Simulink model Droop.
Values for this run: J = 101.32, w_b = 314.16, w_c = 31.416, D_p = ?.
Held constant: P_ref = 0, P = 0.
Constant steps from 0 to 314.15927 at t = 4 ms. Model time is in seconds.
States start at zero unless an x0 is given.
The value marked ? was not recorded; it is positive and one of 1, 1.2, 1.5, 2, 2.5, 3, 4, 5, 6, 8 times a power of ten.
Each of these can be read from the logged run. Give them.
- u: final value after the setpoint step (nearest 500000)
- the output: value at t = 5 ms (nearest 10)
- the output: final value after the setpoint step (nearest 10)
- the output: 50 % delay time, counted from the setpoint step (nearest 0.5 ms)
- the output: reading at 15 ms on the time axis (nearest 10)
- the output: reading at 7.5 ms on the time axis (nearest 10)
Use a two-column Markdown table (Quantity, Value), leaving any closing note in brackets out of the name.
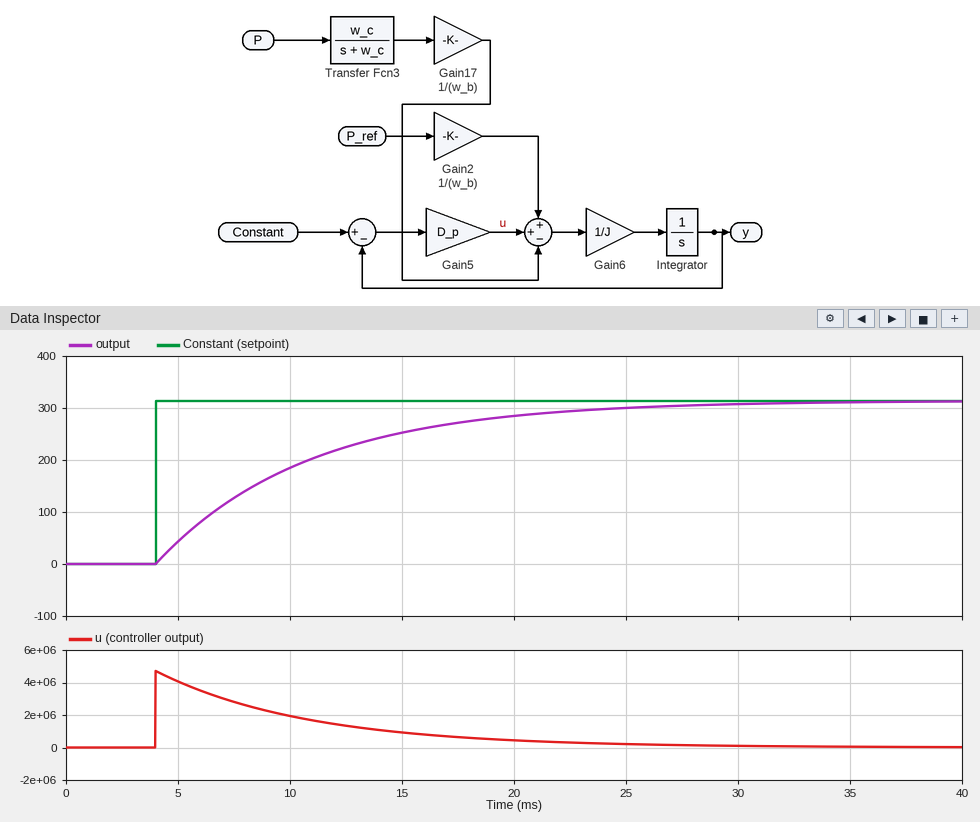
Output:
| Quantity | Value |
|---|---|
| u: final value after the setpoint step | 0 |
| the output: value at t = 5 ms | 40 |
| the output: final value after the setpoint step | 310 |
| the output: 50 % delay time, counted from the setpoint step | 4.5 ms |
| the output: reading at 15 ms on the time axis | 250 |
| the output: reading at 7.5 ms on the time axis | 130 |
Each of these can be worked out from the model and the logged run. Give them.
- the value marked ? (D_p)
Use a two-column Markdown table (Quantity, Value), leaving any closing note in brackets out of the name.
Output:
| Quantity | Value |
|---|---|
| the value marked ? | 15000 |
